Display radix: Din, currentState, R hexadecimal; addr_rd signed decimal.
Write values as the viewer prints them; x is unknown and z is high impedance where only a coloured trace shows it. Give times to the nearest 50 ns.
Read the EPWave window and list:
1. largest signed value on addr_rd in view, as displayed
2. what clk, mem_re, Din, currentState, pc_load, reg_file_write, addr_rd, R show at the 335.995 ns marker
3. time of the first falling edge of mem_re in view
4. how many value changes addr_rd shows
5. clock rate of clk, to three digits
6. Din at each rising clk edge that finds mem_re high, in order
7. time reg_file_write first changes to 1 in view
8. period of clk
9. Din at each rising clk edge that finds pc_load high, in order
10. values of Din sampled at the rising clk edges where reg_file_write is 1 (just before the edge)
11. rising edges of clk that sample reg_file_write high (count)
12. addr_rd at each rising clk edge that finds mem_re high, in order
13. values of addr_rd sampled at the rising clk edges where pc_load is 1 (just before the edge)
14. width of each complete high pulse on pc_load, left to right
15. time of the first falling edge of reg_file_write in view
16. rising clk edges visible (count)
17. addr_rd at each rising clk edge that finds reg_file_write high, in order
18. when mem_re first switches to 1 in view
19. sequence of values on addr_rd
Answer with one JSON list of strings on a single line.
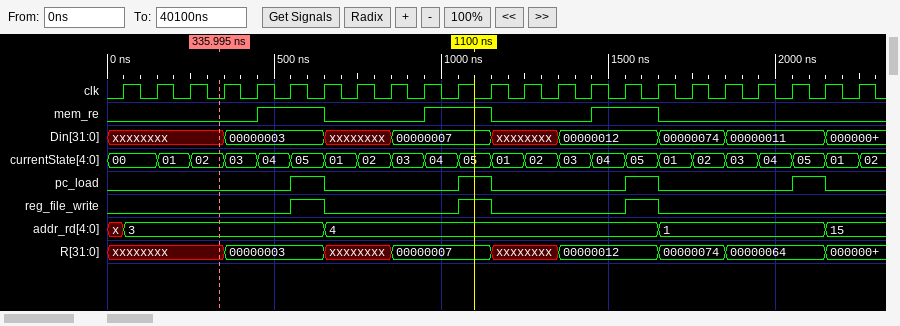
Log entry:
["15", "clk=0, mem_re=0, Din=xxxxxxxx, currentState=02, pc_load=0, reg_file_write=0, addr_rd=3, R=xxxxxxxx", "650 ns", "4", "10.0 MHz", "00000003, 00000003, 00000007, 00000007, 00000012, 00000012", "550 ns", "100 ns", "00000003, 00000007, 00000012, 00000011", "00000003, 00000007, 00000012", "3", "3, 3, 4, 4, 4, 4", "3, 4, 4, 1", "100 ns, 100 ns, 100 ns, 100 ns", "650 ns", "23", "3, 4, 4", "450 ns", "x, 3, 4, 1, 15"]
